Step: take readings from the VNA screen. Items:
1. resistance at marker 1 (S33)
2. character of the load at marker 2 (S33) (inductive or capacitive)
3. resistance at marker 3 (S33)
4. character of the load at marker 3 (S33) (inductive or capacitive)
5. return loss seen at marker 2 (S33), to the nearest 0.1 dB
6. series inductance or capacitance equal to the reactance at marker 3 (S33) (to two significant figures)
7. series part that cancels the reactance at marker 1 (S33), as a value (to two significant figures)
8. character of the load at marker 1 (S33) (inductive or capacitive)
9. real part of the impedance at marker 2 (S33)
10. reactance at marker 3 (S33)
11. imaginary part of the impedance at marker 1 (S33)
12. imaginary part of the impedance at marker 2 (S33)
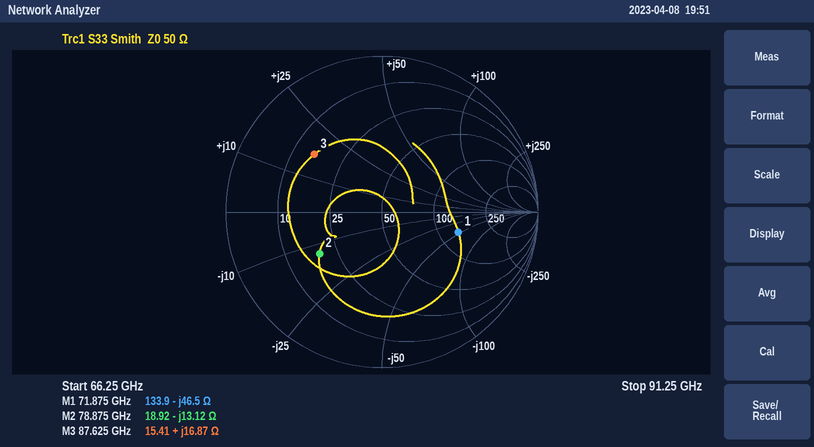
133.9 Ω
capacitive
15.41 Ω
inductive
6.4 dB
31 pH
100 pH
capacitive
18.92 Ω
+16.87 Ω
-46.5 Ω
-13.12 Ω
